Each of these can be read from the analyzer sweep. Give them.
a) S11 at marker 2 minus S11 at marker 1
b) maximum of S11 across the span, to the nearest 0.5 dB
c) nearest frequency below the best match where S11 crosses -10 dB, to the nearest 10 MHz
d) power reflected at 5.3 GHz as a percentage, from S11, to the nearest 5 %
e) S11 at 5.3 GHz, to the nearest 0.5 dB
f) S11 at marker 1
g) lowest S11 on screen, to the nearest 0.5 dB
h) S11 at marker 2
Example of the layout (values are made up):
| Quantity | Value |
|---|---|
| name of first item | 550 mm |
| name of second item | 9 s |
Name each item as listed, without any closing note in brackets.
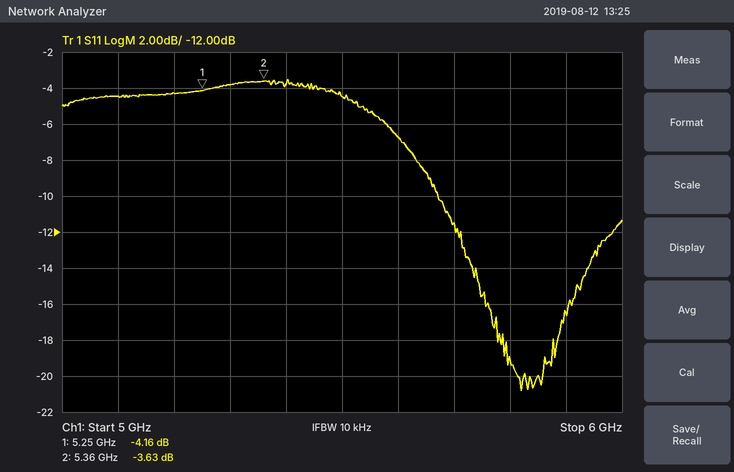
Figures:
| Quantity | Value |
|---|---|
| S11 at marker 2 minus S11 at marker 1 | 0.53 dB |
| maximum of S11 across the span, to the nearest 0.5 dB | -3.5 dB |
| nearest frequency below the best match where S11 crosses -10 dB, to the nearest 10 MHz | 5.67 GHz |
| power reflected at 5.3 GHz as a percentage, from S11, to the nearest 5 % | 40 % |
| S11 at 5.3 GHz, to the nearest 0.5 dB | -4.0 dB |
| S11 at marker 1 | -4.16 dB |
| lowest S11 on screen, to the nearest 0.5 dB | -21.0 dB |
| S11 at marker 2 | -3.63 dB |
